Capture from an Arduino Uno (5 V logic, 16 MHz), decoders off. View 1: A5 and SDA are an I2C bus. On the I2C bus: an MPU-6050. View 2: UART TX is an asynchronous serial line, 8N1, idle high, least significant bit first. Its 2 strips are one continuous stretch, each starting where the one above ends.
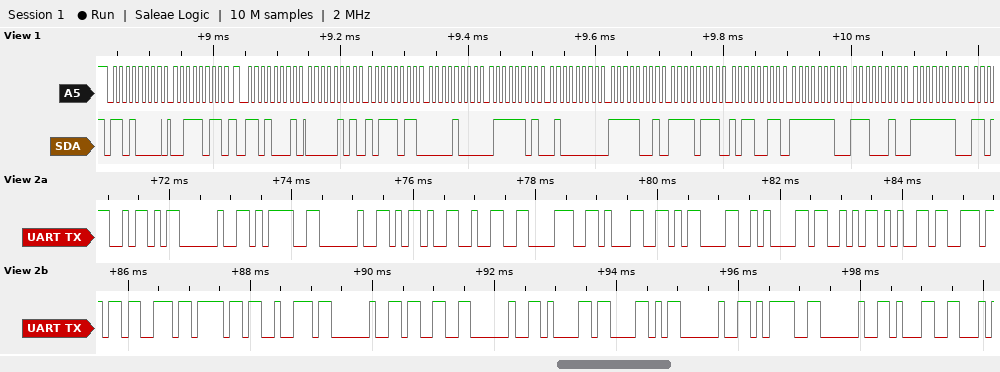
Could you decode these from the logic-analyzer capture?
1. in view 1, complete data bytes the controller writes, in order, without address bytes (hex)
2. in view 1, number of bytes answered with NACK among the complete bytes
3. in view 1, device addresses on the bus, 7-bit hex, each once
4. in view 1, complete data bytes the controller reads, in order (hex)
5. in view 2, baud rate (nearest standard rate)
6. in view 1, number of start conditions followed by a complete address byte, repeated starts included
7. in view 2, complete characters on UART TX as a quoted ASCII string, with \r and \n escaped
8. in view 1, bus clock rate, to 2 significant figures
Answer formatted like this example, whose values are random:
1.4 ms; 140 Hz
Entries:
3B; 0; 0x68; 05 BB 08 7D 40 F9 F7 B3 FE E2 FE; 9600 baud; 2; "Z = -281\r\nSensor 3 aX = 1"; 100 kHz
